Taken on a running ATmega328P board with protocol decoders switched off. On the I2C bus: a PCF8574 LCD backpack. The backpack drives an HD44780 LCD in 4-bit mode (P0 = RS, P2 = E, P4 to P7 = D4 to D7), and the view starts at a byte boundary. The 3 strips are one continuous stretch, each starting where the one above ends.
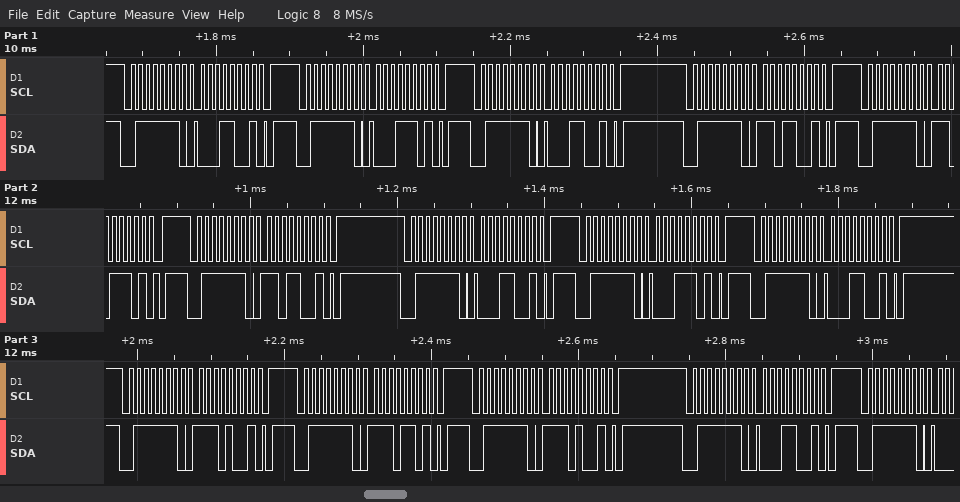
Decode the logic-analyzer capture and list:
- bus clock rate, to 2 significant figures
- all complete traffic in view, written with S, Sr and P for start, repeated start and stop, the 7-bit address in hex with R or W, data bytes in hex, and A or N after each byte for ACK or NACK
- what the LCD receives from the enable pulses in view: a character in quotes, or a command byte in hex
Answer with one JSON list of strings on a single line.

["100 kHz", "S 3FW A 19 A P S 3FW A 1D A P S 3FW A 19 A P S 3FW A D9 A P S 3FW A DD A P S 3FW A D9 A P S 3FW A 19 A P S 3FW A 1D A P S 3FW A 19 A P S 3FW A E9 A P S 3FW A ED A P S 3FW A E9 A P S 3FW A 19 A P S 3FW A", "data 0x1D data 0x1E"]
